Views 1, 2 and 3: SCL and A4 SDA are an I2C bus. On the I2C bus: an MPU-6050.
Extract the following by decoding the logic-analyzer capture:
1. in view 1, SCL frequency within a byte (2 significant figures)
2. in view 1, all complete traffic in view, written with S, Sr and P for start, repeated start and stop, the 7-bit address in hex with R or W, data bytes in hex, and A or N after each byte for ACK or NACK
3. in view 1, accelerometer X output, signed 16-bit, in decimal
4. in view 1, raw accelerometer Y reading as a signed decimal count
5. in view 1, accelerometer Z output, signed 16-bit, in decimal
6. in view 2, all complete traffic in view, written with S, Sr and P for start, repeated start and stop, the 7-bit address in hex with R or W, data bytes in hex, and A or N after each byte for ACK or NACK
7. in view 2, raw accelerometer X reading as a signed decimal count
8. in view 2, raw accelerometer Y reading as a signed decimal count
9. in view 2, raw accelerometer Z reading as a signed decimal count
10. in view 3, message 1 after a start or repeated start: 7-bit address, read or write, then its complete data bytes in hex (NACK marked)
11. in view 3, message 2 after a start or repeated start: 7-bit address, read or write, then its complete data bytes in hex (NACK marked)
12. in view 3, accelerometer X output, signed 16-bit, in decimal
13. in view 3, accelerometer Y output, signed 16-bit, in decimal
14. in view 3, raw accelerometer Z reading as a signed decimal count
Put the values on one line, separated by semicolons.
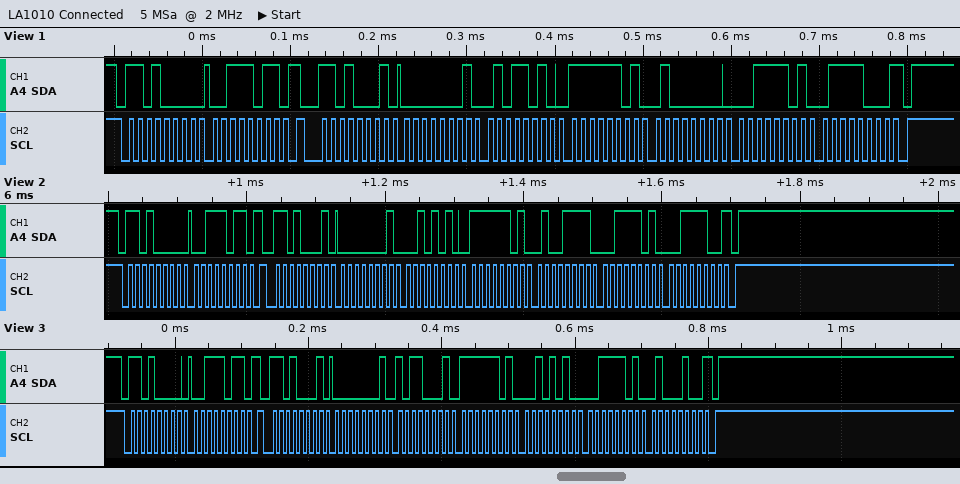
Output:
100 kHz; S 68W A 3B A Sr 68R A 01 A 5A A FD A 40 A 3D A 78 N P; 346; -704; 15736; S 68W A 3B A Sr 68R A 01 A 2A A FD A 4F A 3D A 3C N P; 298; -689; 15676; 0x68 write: 3B; 0x68 read: 01 B1 FD 2A 3D 44 NACK; 433; -726; 15684
